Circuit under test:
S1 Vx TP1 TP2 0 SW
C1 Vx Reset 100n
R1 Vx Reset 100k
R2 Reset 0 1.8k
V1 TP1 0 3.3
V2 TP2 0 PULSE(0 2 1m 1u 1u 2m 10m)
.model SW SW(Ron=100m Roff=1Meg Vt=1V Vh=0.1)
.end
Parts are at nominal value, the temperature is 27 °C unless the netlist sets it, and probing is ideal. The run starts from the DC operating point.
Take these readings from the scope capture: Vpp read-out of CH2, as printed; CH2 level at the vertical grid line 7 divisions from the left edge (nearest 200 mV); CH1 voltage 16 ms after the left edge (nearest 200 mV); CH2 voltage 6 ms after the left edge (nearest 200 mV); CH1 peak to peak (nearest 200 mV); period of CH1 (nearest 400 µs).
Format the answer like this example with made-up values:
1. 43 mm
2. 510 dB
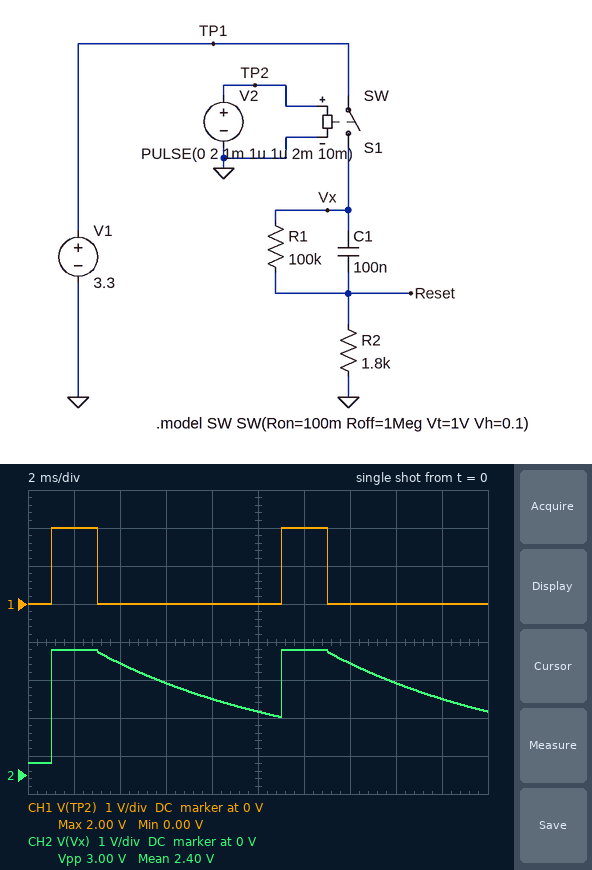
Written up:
1. 3.00 V
2. 3.0 V
3. 0 V
4. 2.4 V
5. 2.0 V
6. 10.0 ms
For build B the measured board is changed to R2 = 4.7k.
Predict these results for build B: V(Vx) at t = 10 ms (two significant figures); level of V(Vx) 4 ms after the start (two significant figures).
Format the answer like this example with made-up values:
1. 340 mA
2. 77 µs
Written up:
1. 1.6 V
2. 2.8 V
